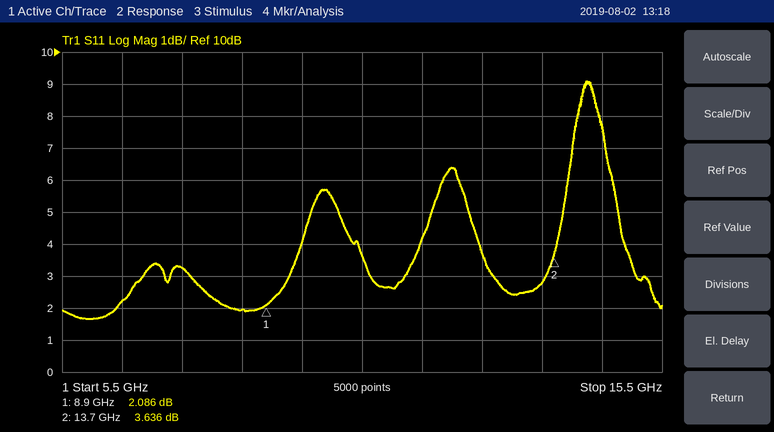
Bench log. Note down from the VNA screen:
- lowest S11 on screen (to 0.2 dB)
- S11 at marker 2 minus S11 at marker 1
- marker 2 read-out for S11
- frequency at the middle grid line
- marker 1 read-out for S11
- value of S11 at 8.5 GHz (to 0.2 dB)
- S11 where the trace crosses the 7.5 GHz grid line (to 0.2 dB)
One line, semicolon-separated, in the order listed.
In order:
1.6 dB; 1.550 dB; 3.636 dB; 10.5 GHz; 2.086 dB; 2.0 dB; 3.2 dB
